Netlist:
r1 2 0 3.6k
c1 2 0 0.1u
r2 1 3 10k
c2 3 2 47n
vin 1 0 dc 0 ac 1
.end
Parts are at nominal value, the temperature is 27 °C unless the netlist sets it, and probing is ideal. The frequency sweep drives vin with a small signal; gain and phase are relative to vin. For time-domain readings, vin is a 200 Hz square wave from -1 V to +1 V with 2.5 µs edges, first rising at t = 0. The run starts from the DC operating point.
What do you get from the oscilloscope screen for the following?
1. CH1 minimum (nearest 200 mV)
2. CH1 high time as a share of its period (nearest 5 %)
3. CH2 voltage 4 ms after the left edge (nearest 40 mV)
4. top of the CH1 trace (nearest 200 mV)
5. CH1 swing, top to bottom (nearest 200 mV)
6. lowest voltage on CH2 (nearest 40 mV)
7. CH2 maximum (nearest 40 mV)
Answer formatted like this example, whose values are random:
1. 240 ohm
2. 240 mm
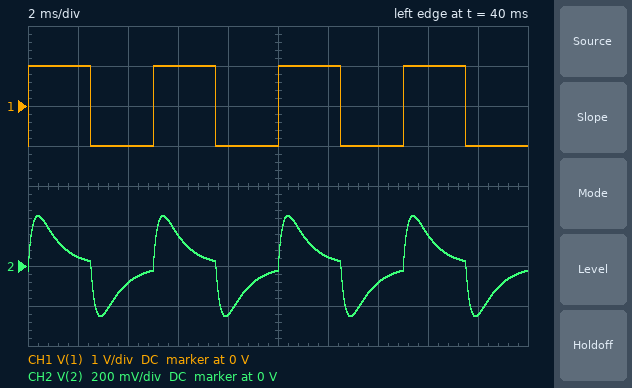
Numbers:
1. -1.0 V
2. 50 %
3. -80 mV
4. 1.0 V
5. 2.0 V
6. -240 mV
7. 240 mV
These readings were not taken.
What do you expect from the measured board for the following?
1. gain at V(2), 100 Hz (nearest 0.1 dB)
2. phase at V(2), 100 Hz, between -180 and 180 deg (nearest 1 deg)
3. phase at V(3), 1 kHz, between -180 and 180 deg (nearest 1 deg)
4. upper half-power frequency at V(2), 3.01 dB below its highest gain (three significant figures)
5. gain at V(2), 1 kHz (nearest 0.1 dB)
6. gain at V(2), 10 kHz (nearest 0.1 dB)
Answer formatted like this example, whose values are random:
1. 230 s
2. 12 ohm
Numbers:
1. -20.5 dB
2. 56 deg
3. -59 deg
4. 1.08 kHz
5. -18.0 dB
6. -36.0 dB
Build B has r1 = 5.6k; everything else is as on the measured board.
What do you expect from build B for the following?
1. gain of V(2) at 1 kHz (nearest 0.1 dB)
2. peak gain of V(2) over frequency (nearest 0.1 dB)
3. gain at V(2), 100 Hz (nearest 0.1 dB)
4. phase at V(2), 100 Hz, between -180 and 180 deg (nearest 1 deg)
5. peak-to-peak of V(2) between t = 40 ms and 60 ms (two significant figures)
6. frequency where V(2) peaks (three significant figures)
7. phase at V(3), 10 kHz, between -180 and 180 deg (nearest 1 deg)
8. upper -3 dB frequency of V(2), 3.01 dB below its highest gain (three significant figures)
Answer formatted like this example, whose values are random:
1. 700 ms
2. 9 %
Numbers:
1. -17.5 dB
2. -13.8 dB
3. -17.3 dB
4. 48 deg
5. 570 mV
6. 310 Hz
7. -87 deg
8. 890 Hz
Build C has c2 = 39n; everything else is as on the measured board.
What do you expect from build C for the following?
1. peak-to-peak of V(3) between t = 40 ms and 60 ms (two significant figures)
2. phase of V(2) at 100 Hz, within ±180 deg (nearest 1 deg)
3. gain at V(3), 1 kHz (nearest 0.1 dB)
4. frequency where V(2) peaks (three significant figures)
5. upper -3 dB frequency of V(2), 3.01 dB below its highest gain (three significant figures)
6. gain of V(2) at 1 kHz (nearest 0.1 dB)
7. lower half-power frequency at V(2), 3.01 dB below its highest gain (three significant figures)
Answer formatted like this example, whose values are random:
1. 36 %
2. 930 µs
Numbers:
1. 2.0 V
2. 59 deg
3. -6.8 dB
4. 425 Hz
5. 1.16 kHz
6. -18.2 dB
7. 155 Hz
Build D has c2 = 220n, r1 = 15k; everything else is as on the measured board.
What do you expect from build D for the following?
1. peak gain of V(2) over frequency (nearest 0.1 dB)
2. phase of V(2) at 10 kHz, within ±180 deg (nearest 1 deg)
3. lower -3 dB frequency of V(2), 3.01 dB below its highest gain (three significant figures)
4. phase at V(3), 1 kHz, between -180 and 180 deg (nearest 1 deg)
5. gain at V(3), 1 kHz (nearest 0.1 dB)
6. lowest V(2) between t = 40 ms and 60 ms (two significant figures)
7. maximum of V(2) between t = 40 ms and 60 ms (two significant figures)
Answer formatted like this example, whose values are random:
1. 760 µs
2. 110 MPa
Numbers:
1. -6.5 dB
2. -88 deg
3. 21.4 Hz
4. -73 deg
5. -13.1 dB
6. -470 mV
7. 470 mV
